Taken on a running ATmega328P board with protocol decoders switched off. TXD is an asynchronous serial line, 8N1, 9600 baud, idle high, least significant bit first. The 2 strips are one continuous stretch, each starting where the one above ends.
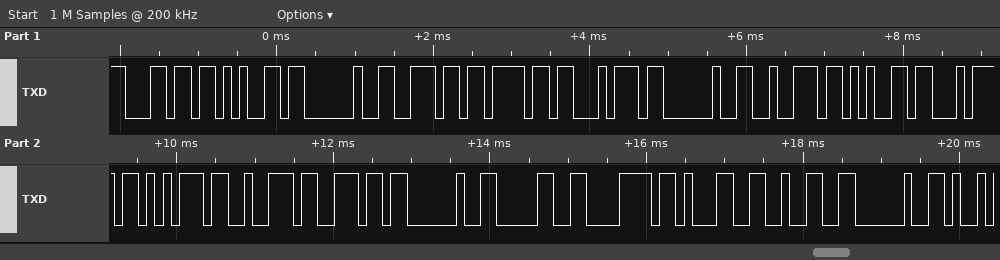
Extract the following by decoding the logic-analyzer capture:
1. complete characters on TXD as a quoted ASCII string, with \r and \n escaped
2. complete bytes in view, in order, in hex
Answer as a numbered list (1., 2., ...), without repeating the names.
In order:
1. "le not return 0x12 "
2. 6C 65 20 6E 6F 74 20 72 65 74 75 72 6E 20 30 78 31 32 20
